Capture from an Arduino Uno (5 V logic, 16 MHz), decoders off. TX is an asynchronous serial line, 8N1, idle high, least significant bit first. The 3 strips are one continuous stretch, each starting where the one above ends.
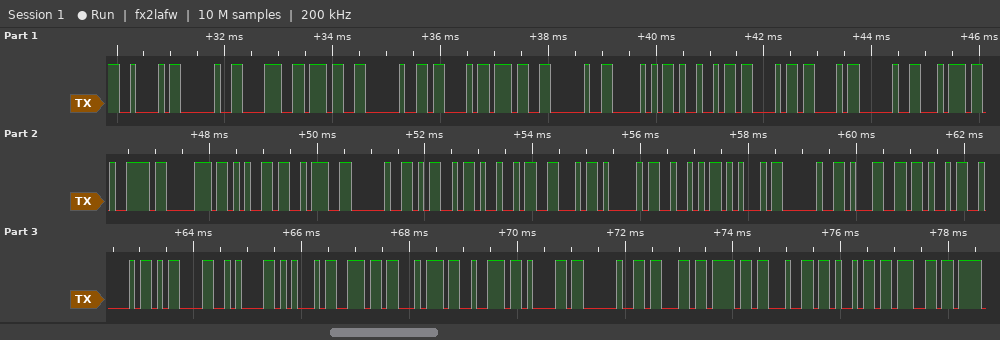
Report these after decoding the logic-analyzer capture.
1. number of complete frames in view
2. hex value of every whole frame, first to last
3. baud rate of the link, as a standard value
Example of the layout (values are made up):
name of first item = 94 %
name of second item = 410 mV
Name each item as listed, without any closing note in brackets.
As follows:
number of complete frames in view = 42
hex value of every whole frame, first to last = 0x42 0x20 0x38 0x37 0x20 0x43 0x37 0x20 0x50 0x49 0x43 0x43 0x20 0x74 0x79 0x70 0x65 0x3A 0x20 0x4D 0x49 0x46 0x41 0x52 0x45 0x20 0x31 0x4B 0x42 0x0D 0x0A 0x45 0x6E 0x74 0x72 0x61 0x20 0x63 0x6F 0x64 0x69 0x67
baud rate of the link, as a standard value = 9600 baud
